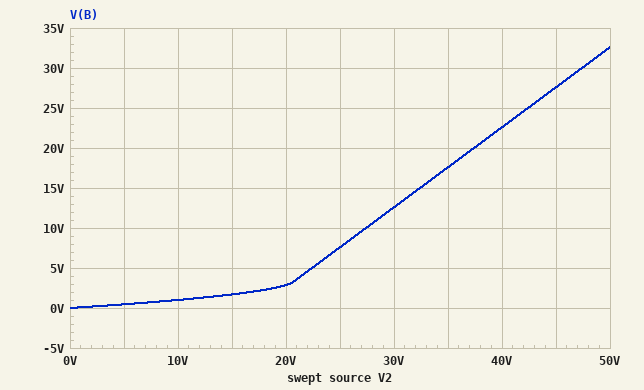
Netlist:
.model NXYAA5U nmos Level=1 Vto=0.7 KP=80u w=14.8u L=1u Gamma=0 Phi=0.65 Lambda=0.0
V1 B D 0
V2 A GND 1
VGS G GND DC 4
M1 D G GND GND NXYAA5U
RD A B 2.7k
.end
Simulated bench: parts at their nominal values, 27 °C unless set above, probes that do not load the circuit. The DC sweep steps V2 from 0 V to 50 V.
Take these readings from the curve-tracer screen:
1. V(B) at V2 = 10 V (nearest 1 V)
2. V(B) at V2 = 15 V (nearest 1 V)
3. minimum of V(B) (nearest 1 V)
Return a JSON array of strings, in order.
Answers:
["1 V", "2 V", "0 V"]
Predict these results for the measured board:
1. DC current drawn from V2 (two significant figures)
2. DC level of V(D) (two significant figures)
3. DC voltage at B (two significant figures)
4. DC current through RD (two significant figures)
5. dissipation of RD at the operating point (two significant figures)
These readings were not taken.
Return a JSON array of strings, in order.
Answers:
["340 µA", "88 mV", "88 mV", "340 µA", "310 µW"]
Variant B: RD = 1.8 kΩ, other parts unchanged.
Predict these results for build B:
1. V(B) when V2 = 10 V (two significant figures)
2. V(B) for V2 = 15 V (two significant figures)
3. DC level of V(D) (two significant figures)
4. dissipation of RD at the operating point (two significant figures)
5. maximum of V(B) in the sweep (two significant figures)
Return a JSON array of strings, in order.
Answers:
["1.6 V", "3.4 V", "130 mV", "420 µW", "38 V"]
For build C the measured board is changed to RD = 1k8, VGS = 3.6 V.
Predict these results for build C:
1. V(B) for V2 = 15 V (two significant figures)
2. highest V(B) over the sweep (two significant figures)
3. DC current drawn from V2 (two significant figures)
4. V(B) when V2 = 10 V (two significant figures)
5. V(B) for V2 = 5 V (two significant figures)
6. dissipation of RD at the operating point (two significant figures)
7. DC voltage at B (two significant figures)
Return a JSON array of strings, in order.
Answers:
["6.0 V", "41 V", "480 µA", "2.0 V", "790 mV", "410 µW", "140 mV"]
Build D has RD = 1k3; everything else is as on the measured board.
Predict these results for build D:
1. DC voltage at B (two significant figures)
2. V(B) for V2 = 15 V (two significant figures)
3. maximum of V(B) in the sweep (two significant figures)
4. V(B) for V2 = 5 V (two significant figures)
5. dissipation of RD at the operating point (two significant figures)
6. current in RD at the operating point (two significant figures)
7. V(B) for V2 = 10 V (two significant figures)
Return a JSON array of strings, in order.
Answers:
["170 mV", "6.6 V", "42 V", "930 mV", "530 µW", "640 µA", "2.3 V"]
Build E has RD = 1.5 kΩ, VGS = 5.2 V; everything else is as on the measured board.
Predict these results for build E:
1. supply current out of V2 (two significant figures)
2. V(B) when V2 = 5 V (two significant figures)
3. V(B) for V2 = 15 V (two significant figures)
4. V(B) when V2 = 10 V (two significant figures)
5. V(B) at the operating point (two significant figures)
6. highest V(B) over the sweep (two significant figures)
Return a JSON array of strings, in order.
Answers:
["590 µA", "590 mV", "2.1 V", "1.3 V", "110 mV", "32 V"]
